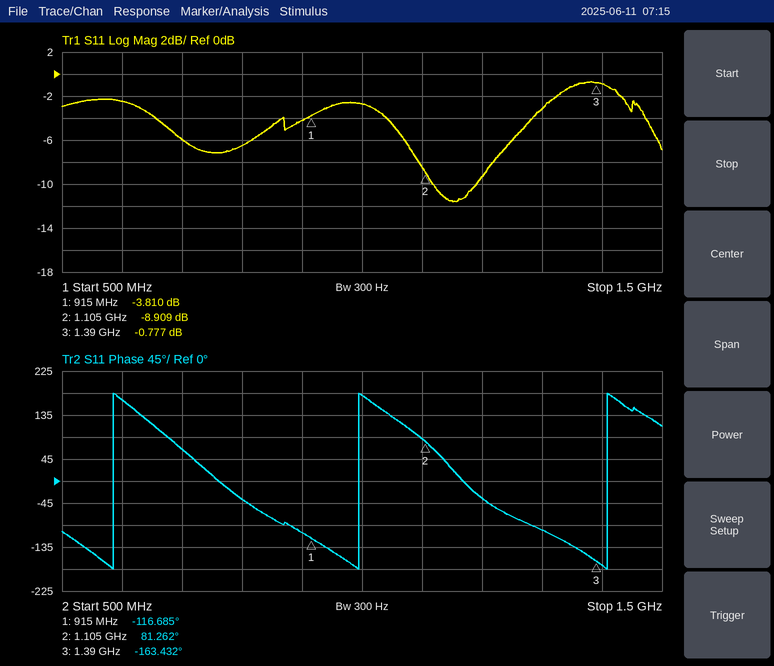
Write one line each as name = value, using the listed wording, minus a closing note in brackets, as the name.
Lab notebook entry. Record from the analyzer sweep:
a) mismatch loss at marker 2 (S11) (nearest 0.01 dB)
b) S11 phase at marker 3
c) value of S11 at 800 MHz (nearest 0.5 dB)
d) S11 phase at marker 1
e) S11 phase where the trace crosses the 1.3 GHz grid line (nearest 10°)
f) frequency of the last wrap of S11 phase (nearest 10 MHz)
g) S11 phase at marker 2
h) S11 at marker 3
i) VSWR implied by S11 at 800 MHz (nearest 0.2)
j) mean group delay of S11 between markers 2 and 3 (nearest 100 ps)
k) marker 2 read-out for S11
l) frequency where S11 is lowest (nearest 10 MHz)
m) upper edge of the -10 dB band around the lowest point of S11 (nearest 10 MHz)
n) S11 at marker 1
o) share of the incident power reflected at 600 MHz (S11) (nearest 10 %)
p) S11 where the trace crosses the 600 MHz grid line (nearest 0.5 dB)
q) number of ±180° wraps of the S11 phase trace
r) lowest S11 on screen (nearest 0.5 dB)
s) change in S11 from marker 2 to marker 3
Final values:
mismatch loss at marker 2 (S11) = 0.60 dB
S11 phase at marker 3 = -163.432°
value of S11 at 800 MHz = -6.5 dB
S11 phase at marker 1 = -116.685°
S11 phase where the trace crosses the 1.3 GHz grid line = -100°
frequency of the last wrap of S11 phase = 1.41 GHz
S11 phase at marker 2 = 81.262°
S11 at marker 3 = -0.777 dB
VSWR implied by S11 at 800 MHz = 2.8
mean group delay of S11 between markers 2 and 3 = 2.4 ns
marker 2 read-out for S11 = -8.909 dB
frequency where S11 is lowest = 1.15 GHz
upper edge of the -10 dB band around the lowest point of S11 = 1.19 GHz
S11 at marker 1 = -3.810 dB
share of the incident power reflected at 600 MHz (S11) = 60 %
S11 where the trace crosses the 600 MHz grid line = -2.5 dB
number of ±180° wraps of the S11 phase trace = 3
lowest S11 on screen = -11.5 dB
change in S11 from marker 2 to marker 3 = 8.132 dB
